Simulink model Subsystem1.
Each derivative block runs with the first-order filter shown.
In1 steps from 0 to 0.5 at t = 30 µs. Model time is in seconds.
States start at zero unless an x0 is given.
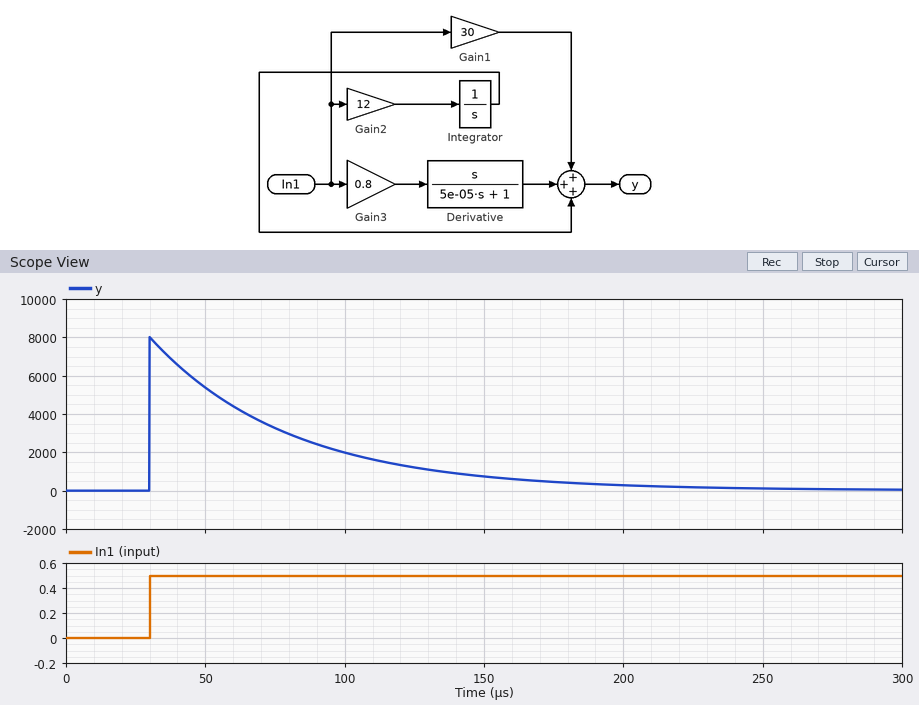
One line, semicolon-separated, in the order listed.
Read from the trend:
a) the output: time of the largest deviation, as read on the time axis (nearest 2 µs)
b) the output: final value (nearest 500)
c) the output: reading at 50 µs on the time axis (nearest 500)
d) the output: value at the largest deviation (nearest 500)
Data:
30 µs; 0; 5500; 8000
